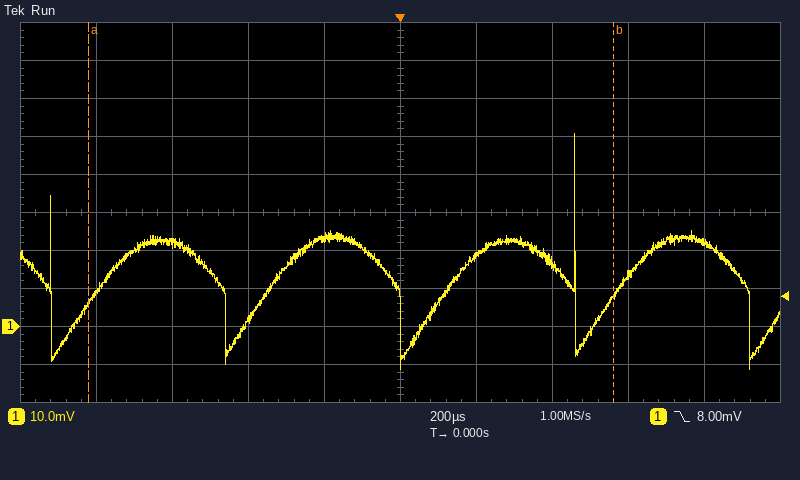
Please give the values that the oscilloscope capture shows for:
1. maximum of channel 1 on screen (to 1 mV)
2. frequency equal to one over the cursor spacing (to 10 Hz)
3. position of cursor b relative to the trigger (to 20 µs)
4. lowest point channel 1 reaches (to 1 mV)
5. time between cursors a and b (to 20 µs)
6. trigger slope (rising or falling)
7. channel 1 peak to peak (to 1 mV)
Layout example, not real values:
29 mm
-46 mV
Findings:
51 mV
720 Hz
+560 µs
-11 mV
1.38 ms
falling
62 mV
